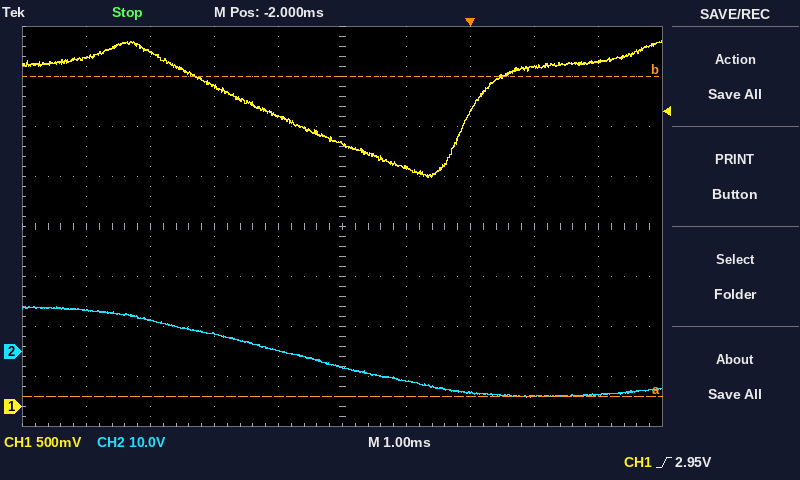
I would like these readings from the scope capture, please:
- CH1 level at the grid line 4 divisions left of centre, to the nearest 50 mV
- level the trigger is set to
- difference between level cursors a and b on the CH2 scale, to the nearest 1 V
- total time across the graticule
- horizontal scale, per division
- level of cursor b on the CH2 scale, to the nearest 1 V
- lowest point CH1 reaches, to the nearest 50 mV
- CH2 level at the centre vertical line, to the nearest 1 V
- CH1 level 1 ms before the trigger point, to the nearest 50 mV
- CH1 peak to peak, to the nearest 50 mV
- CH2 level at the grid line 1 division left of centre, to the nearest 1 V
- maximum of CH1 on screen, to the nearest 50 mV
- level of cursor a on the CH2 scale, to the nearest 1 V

3.50 V
2.95 V
64 V
10 ms
1 ms
55 V
2.30 V
-3 V
2.40 V
1.35 V
0 V
3.65 V
-9 V
